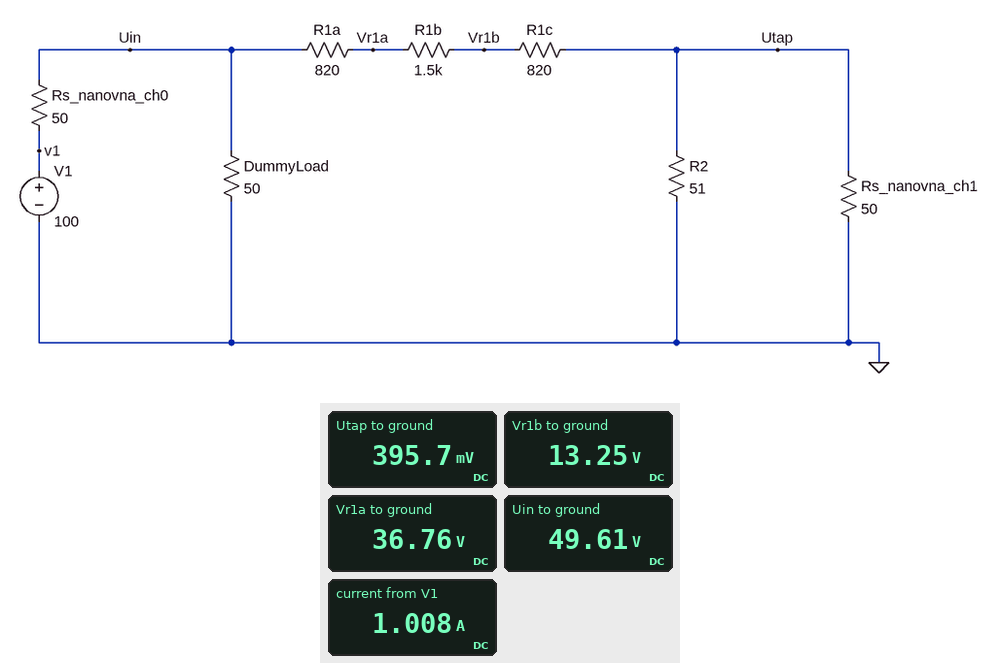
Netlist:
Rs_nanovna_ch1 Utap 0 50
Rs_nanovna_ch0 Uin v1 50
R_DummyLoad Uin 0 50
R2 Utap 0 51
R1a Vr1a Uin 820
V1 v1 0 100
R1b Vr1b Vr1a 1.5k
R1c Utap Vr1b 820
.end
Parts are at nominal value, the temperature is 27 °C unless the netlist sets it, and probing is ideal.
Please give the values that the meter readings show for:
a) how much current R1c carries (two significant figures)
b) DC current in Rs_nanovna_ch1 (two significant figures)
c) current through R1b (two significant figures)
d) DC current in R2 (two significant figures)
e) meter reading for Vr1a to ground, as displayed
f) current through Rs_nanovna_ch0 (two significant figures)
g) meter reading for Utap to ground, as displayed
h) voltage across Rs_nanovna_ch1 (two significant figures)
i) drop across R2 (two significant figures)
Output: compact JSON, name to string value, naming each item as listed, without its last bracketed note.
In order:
{"how much current R1c carries": "16 mA", "DC current in Rs_nanovna_ch1": "7.9 mA", "current through R1b": "16 mA", "DC current in R2": "7.8 mA", "meter reading for Vr1a to ground, as displayed": "36.76 V", "current through Rs_nanovna_ch0": "1.0 A", "meter reading for Utap to ground, as displayed": "395.7 mV", "voltage across Rs_nanovna_ch1": "400 mV", "drop across R2": "400 mV"}
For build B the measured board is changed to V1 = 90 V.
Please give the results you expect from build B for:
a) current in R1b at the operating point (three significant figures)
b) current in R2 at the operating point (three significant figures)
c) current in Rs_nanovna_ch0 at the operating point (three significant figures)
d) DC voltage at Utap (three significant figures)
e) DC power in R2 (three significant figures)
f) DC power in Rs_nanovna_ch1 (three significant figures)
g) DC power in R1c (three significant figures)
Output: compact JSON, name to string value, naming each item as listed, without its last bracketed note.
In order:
{"current in R1b at the operating point": "14.1 mA", "current in R2 at the operating point": "6.98 mA", "current in Rs_nanovna_ch0 at the operating point": "907 mA", "DC voltage at Utap": "356 mV", "DC power in R2": "2.49 mW", "DC power in Rs_nanovna_ch1": "2.54 mW", "DC power in R1c": "163 mW"}
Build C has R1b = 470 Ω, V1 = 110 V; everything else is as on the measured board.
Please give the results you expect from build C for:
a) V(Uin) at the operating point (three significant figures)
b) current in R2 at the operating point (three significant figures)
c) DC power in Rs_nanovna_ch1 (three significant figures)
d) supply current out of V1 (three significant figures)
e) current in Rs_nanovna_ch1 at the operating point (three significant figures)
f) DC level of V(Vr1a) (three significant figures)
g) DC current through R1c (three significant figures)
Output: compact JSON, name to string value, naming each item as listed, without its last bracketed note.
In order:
{"V(Uin) at the operating point": "54.4 V", "current in R2 at the operating point": "12.6 mA", "DC power in Rs_nanovna_ch1": "8.26 mW", "supply current out of V1": "1.11 A", "current in Rs_nanovna_ch1 at the operating point": "12.9 mA", "DC level of V(Vr1a)": "33.5 V", "DC current through R1c": "25.5 mA"}
